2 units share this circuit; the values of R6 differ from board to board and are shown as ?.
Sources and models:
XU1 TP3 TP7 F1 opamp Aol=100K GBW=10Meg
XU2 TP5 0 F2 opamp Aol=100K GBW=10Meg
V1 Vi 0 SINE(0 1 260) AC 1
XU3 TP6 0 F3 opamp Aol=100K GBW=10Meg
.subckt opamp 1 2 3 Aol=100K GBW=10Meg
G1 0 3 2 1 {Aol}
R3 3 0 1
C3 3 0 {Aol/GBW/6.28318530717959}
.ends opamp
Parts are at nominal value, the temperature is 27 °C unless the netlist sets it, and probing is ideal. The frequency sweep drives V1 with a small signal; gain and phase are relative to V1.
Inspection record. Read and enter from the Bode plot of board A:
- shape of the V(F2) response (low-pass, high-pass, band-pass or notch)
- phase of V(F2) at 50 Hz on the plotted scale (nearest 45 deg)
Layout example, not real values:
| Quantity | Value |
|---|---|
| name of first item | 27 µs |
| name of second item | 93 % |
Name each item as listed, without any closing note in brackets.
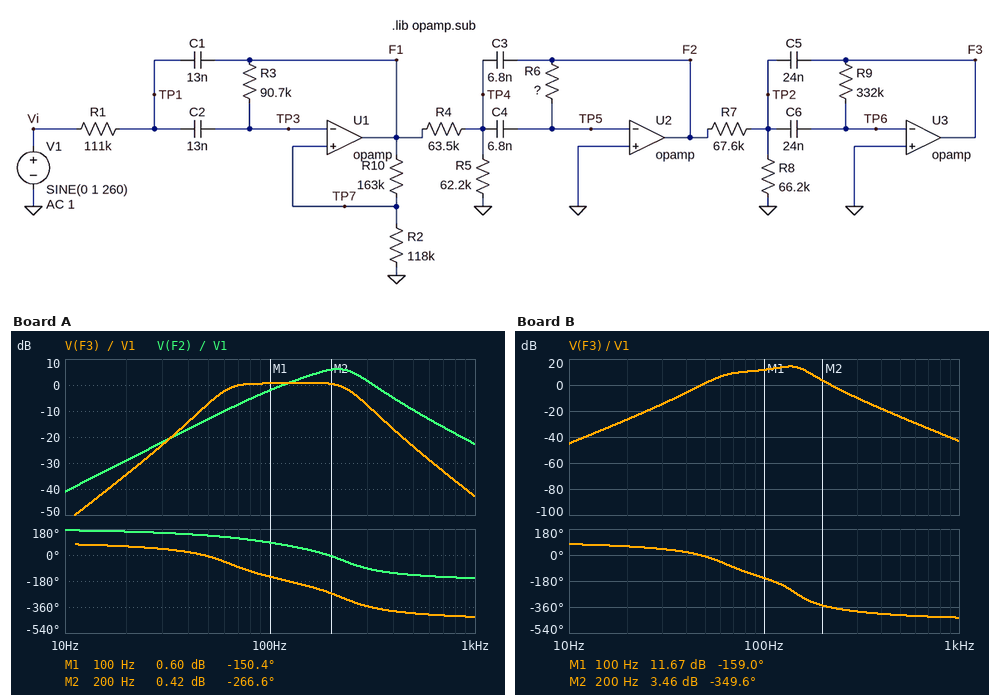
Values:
| Quantity | Value |
|---|---|
| shape of the V(F2) response | band-pass |
| phase of V(F2) at 50 Hz on the plotted scale | 135 deg |
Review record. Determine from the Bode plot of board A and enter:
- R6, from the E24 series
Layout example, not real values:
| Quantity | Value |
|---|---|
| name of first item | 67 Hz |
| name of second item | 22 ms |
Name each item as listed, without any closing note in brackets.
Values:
| Quantity | Value |
|---|---|
| R6, from the E24 series | 330 kΩ |
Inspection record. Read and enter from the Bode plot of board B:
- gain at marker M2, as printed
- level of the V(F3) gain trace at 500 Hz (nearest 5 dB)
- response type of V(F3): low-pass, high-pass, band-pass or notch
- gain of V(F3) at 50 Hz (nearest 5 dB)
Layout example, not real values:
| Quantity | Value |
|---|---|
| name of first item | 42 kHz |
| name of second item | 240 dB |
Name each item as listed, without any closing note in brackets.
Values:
| Quantity | Value |
|---|---|
| gain at marker M2, as printed | 3.46 dB |
| level of the V(F3) gain trace at 500 Hz | -25 dB |
| response type of V(F3): low-pass, high-pass, band-pass or notch | band-pass |
| gain of V(F3) at 50 Hz | 0 dB |
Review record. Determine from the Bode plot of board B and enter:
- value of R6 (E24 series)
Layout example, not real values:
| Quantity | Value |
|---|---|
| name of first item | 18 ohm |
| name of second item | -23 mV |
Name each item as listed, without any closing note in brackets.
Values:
| Quantity | Value |
|---|---|
| value of R6 | 820 kΩ |
